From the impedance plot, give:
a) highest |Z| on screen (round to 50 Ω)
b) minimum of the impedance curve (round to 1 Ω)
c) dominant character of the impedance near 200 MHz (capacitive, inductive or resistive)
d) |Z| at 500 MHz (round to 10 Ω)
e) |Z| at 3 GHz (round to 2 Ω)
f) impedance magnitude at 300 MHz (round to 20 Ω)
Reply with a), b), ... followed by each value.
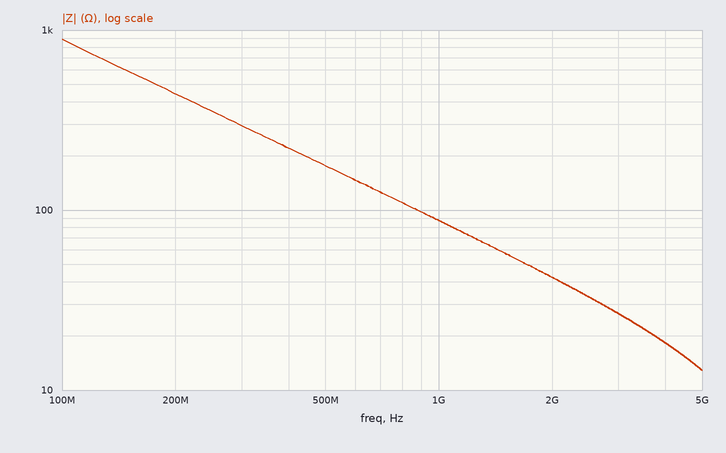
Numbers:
a) 900 Ω
b) 13 Ω
c) capacitive
d) 180 Ω
e) 26 Ω
f) 300 Ω
